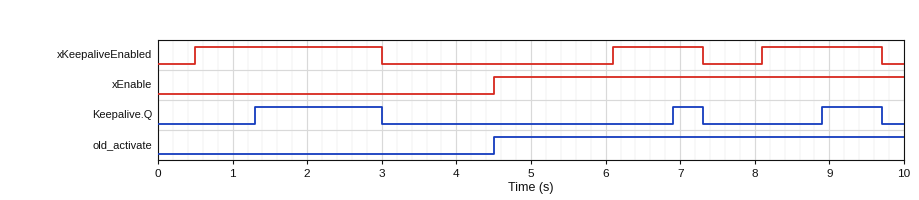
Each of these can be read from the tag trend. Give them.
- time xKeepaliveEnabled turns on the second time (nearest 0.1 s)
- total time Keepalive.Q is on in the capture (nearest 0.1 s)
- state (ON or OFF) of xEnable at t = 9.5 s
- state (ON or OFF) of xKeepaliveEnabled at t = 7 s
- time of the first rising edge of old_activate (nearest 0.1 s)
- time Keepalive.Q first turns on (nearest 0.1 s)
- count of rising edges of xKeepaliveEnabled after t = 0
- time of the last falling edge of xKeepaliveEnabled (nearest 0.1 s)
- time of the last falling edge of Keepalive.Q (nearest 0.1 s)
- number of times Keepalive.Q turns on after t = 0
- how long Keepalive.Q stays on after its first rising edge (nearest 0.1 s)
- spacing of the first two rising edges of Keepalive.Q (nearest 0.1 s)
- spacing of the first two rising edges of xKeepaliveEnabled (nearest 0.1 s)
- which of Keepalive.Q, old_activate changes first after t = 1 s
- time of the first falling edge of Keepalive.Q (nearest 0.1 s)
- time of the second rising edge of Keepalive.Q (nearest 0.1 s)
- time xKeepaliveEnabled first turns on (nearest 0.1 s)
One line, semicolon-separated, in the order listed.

6.1 s; 2.9 s; ON; ON; 4.5 s; 1.3 s; 3; 9.7 s; 9.7 s; 3; 1.7 s; 5.6 s; 5.6 s; Keepalive.Q; 3.0 s; 6.9 s; 0.5 s
